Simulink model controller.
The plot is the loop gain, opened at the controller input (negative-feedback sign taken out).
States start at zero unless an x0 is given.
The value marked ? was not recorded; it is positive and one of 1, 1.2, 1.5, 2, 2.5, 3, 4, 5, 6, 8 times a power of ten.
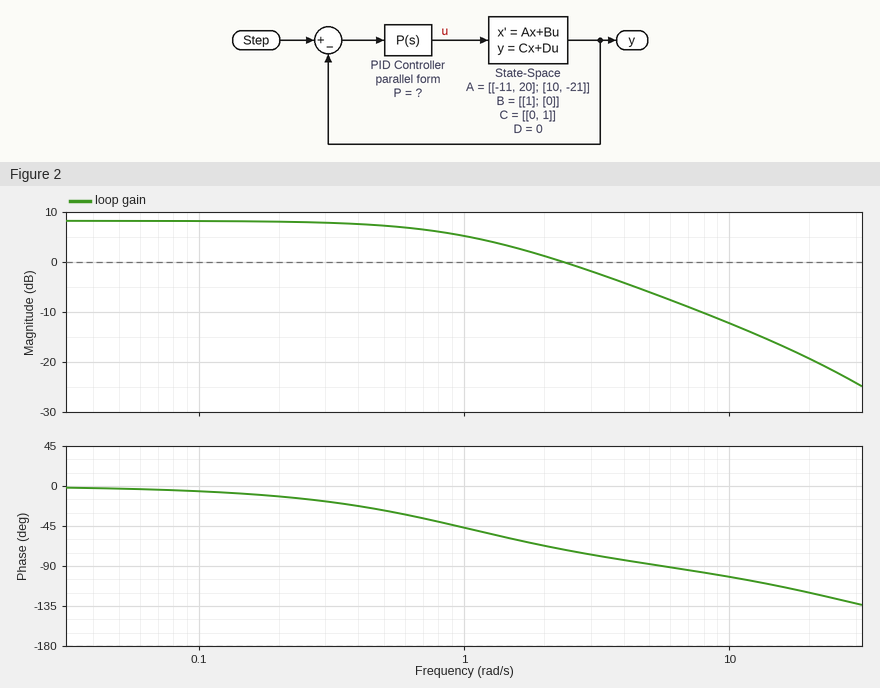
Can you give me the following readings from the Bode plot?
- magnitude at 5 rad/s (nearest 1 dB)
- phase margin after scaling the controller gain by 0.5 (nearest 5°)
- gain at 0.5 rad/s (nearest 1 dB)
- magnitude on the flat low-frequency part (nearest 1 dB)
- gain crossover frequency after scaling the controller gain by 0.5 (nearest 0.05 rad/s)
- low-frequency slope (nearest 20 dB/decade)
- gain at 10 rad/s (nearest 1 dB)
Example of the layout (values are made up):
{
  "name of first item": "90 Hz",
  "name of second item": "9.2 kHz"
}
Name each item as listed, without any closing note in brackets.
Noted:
{
  "magnitude at 5 rad/s": "-6 dB",
  "phase margin after scaling the controller gain by 0.5": "140°",
  "gain at 0.5 rad/s": "7 dB",
  "magnitude on the flat low-frequency part": "8 dB",
  "gain crossover frequency after scaling the controller gain by 0.5": "0.80 rad/s",
  "low-frequency slope": "0 dB/decade",
  "gain at 10 rad/s": "-12 dB"
}
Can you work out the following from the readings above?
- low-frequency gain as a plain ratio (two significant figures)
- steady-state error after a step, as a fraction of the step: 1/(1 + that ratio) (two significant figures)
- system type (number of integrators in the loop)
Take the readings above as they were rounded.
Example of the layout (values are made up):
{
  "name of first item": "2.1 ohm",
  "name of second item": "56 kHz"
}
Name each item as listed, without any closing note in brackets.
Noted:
{
  "low-frequency gain as a plain ratio": "2.5",
  "steady-state error after a step, as a fraction of the step: 1/(1 + that ratio)": "0.29",
  "system type": "0"
}
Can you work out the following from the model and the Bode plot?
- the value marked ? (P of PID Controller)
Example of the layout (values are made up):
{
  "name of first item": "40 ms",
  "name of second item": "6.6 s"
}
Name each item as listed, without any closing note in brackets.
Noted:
{
  "the value marked ?": "8"
}
